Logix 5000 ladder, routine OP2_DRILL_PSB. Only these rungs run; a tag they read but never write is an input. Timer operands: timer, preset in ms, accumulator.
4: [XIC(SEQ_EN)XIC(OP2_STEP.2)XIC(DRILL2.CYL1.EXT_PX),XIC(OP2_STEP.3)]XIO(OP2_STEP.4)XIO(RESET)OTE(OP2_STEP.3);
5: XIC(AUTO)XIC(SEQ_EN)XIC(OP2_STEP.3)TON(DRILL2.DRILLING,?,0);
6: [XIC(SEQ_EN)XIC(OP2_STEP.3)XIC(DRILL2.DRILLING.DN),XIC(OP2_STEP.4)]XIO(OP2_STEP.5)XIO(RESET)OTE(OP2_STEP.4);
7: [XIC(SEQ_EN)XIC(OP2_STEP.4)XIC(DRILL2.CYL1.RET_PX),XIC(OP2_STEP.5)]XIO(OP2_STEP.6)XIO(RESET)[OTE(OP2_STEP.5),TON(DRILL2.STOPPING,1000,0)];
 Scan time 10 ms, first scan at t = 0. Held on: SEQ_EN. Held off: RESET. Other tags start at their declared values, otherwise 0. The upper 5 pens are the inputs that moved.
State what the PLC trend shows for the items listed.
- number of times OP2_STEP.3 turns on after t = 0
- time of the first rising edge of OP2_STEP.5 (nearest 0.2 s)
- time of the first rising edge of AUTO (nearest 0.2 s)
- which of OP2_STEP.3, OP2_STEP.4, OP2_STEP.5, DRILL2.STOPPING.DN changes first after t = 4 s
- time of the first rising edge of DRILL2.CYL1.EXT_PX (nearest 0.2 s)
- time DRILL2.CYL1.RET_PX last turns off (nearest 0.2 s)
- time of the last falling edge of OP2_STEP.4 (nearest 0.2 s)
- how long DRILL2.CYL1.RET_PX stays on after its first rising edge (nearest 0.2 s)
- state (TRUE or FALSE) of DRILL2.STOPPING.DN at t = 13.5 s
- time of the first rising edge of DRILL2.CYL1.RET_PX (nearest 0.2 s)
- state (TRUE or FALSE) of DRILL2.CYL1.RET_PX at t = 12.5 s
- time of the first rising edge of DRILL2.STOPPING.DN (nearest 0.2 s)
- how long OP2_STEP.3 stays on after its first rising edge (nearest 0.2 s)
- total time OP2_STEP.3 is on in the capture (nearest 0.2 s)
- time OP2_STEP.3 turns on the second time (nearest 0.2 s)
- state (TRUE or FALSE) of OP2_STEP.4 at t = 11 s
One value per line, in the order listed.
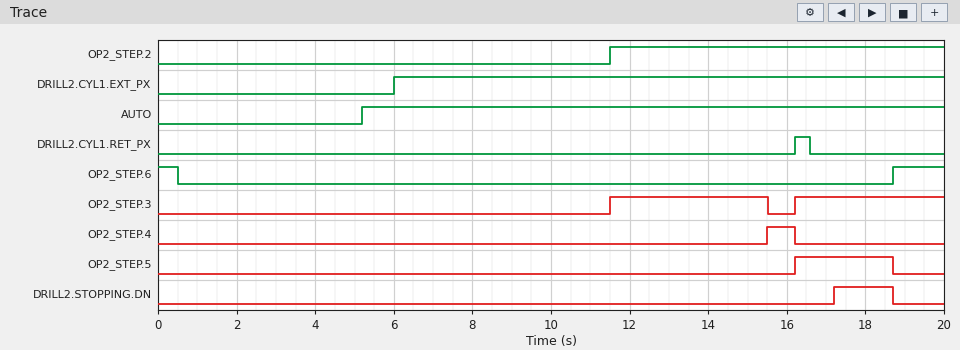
2
16.2 s
5.2 s
OP2_STEP.3
6.0 s
16.6 s
16.2 s
0.4 s
FALSE
16.2 s
FALSE
17.2 s
4.0 s
7.8 s
16.2 s
FALSE
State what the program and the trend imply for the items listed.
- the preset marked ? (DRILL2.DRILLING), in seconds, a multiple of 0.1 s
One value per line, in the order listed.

4.0 s
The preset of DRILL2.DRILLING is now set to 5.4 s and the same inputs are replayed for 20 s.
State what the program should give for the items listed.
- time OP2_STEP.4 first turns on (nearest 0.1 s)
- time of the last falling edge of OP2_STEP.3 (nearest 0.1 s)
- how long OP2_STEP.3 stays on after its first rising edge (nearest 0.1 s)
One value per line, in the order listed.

16.9 s
16.9 s
5.4 s
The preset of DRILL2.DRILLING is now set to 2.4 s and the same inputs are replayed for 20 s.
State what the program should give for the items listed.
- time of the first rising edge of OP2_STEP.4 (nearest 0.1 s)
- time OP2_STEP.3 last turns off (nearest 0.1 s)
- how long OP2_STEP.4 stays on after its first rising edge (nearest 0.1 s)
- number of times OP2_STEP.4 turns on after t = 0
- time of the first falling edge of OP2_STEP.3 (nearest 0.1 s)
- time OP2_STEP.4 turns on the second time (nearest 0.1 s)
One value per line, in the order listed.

13.9 s
18.7 s
2.3 s
2
13.9 s
18.7 s
